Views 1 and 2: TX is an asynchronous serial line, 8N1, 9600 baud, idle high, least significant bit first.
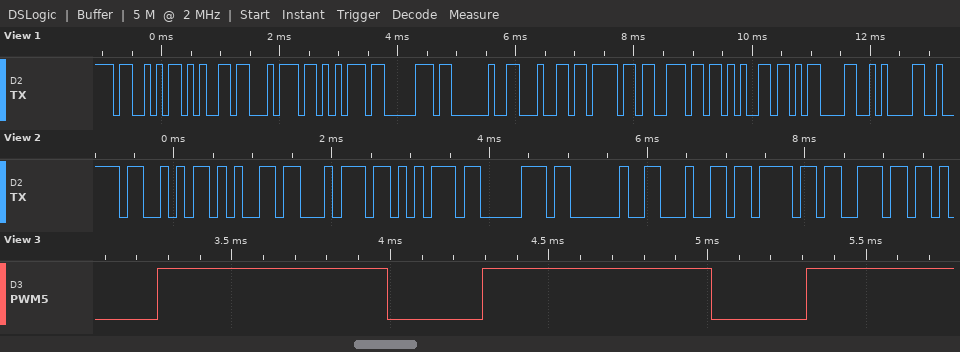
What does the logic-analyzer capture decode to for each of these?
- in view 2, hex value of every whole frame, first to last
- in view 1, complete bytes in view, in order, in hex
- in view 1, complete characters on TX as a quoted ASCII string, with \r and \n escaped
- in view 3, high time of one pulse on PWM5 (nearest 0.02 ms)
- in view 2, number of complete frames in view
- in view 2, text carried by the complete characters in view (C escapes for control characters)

0x53 0x65 0x74 0x75 0x70 0x20 0x64 0x6F 0x6E
0x53 0x65 0x74 0x75 0x70 0x20 0x64 0x6F 0x6E 0x65 0x0D 0x0A
"Setup done\r\n"
0.72 ms
9
"Setup don"
